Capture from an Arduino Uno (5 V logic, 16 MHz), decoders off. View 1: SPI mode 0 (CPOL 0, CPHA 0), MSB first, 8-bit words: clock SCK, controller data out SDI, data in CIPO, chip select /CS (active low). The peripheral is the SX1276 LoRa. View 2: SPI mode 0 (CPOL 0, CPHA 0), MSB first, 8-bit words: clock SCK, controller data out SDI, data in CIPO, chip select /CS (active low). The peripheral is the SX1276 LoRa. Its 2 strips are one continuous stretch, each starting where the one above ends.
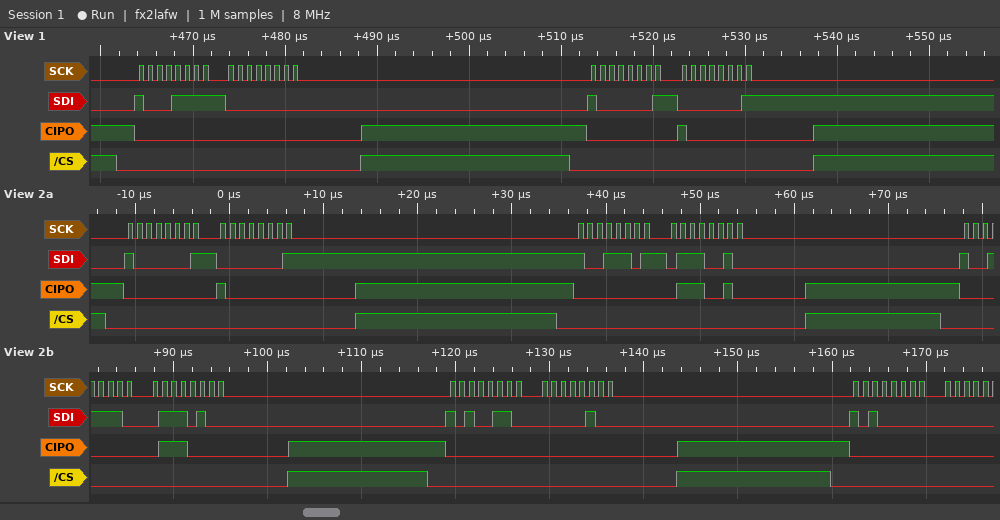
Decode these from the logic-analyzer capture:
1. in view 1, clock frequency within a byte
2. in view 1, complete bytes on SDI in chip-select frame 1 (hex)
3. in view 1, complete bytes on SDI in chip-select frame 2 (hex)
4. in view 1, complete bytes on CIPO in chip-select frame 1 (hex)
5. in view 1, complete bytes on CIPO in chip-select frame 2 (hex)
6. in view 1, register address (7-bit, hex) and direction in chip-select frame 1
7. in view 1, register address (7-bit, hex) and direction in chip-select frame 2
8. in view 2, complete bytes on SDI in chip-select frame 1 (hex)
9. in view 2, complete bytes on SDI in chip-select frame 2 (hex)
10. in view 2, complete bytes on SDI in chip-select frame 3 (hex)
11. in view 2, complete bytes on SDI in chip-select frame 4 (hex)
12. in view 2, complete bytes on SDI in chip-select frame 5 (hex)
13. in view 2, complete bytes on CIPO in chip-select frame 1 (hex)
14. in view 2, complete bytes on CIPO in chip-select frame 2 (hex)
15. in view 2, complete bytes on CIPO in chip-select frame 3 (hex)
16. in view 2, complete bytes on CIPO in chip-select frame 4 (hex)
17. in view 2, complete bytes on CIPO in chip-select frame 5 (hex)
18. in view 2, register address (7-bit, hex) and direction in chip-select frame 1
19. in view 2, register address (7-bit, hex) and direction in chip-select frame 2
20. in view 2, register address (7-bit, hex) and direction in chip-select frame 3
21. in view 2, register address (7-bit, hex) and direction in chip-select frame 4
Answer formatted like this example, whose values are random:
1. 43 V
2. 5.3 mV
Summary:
1. 1 MHz
2. 8F 00
3. 81 01
4. 00 00
5. 00 80
6. 0x0F write
7. 0x01 write
8. 0x81 0x01
9. 0x9D 0x72
10. 0x9E 0x74
11. 0xA6 0x04
12. 0xA0
13. 0x00 0x80
14. 0x00 0x72
15. 0x00 0x70
16. 0x00 0x00
17. 0x00
18. 0x01 write
19. 0x1D write
20. 0x1E write
21. 0x26 write
